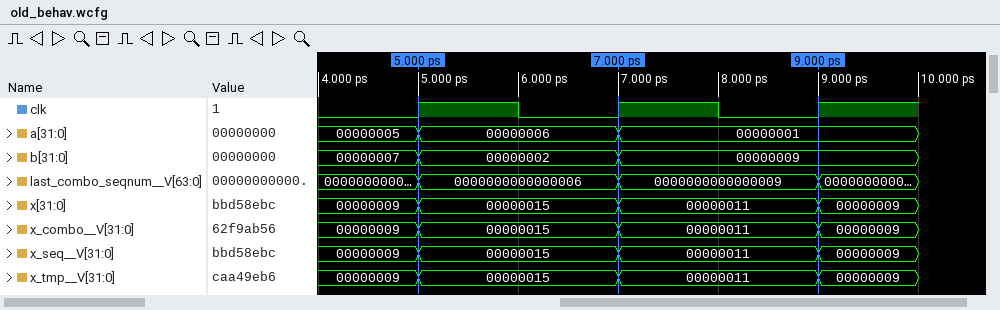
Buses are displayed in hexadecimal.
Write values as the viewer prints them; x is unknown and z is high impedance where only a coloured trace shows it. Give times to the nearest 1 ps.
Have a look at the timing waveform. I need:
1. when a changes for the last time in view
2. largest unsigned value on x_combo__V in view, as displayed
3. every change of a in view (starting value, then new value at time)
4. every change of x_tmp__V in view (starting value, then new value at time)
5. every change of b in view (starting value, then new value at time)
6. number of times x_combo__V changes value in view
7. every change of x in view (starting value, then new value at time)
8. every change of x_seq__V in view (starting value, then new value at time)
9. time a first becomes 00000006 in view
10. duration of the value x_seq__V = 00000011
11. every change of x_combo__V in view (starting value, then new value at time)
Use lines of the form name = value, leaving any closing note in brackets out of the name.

when a changes for the last time in view = 7 ps
largest unsigned value on x_combo__V in view, as displayed = 00000015
every change of a in view = 00000005, 00000006 at 5 ps, 00000001 at 7 ps
every change of x_tmp__V in view = 00000009, 00000015 at 5 ps, 00000011 at 7 ps, 00000009 at 9 ps
every change of b in view = 00000007, 00000002 at 5 ps, 00000009 at 7 ps
number of times x_combo__V changes value in view = 3
every change of x in view = 00000009, 00000015 at 5 ps, 00000011 at 7 ps, 00000009 at 9 ps
every change of x_seq__V in view = 00000009, 00000015 at 5 ps, 00000011 at 7 ps, 00000009 at 9 ps
time a first becomes 00000006 in view = 5 ps
duration of the value x_seq__V = 00000011 = 2 ps
every change of x_combo__V in view = 00000009, 00000015 at 5 ps, 00000011 at 7 ps, 00000009 at 9 ps
